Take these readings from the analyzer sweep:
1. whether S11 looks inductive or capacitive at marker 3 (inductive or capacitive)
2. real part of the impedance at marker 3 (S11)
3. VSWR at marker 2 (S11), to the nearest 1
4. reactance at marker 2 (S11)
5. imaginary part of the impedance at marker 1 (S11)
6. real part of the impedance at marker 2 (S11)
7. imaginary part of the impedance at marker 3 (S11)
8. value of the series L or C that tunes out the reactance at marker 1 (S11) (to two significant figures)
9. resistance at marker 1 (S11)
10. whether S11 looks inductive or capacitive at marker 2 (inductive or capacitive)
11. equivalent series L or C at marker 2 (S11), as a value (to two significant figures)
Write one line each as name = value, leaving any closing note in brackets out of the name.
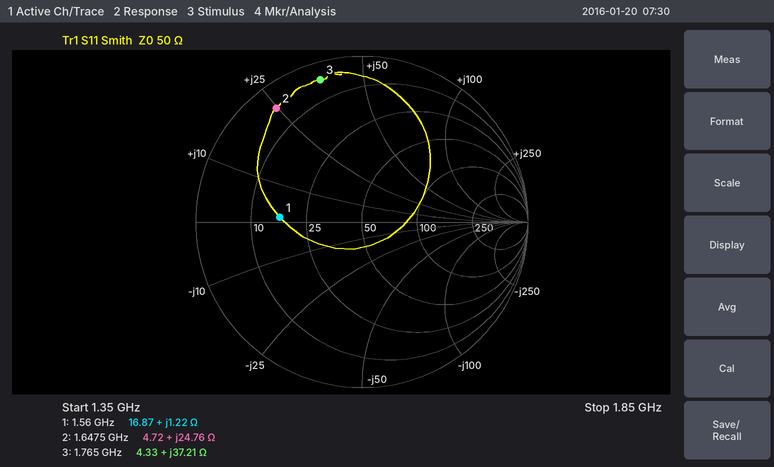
whether S11 looks inductive or capacitive at marker 3 = inductive
real part of the impedance at marker 3 = 4.33 Ω
VSWR at marker 2 (S11), to the nearest 1 = 13
reactance at marker 2 = +24.76 Ω
imaginary part of the impedance at marker 1 = +1.22 Ω
real part of the impedance at marker 2 = 4.72 Ω
imaginary part of the impedance at marker 3 = +37.21 Ω
value of the series L or C that tunes out the reactance at marker 1 (S11) = 84 pF
resistance at marker 1 = 16.87 Ω
whether S11 looks inductive or capacitive at marker 2 = inductive
equivalent series L or C at marker 2 (S11), as a value = 2.4 nH
